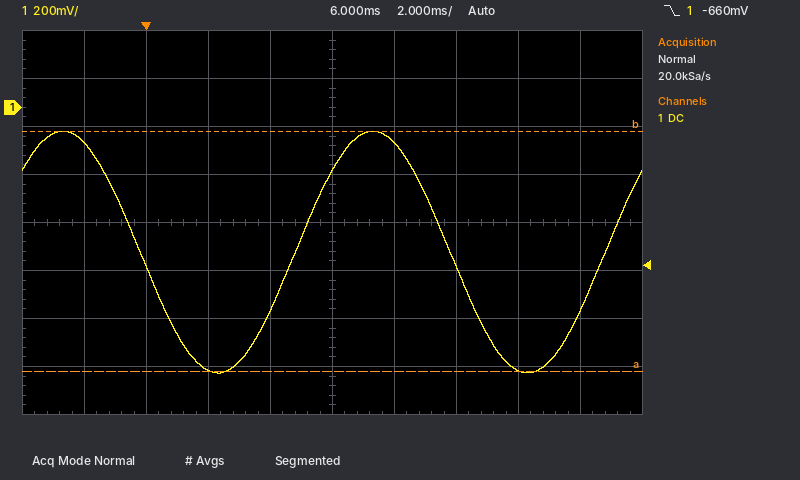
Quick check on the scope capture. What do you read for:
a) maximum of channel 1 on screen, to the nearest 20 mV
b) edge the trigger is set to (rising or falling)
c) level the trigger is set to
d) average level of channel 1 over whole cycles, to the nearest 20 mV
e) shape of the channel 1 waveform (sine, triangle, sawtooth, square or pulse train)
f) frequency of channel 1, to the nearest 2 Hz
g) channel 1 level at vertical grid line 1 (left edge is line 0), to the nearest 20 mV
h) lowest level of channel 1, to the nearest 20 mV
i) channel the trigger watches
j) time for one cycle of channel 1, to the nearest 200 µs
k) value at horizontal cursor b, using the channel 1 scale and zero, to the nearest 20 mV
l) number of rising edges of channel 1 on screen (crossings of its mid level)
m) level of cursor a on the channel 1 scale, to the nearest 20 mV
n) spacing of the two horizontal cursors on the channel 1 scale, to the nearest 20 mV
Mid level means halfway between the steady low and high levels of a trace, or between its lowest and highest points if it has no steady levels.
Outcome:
-100 mV
falling
-660 mV
-600 mV
sine
100 Hz
-140 mV
-1.10 V
channel 1
10.0 ms
-100 mV
2
-1.10 V
1.00 V
